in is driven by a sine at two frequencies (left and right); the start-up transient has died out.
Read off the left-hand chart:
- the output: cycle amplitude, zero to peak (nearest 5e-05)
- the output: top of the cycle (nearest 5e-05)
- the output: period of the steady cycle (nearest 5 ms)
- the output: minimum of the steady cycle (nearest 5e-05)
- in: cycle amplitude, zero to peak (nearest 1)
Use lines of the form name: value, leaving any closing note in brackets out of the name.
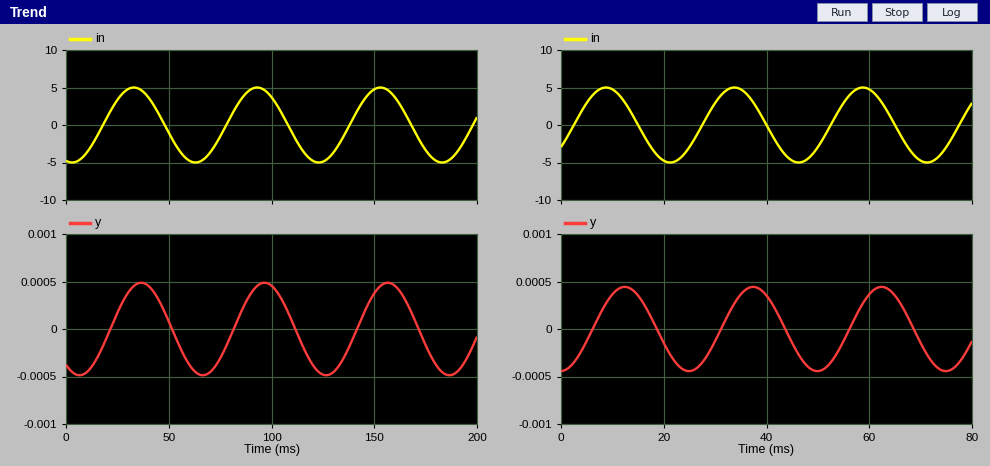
the output: cycle amplitude, zero to peak: 0.00050
the output: top of the cycle: 0.00050
the output: period of the steady cycle: 60 ms
the output: minimum of the steady cycle: -0.00050
in: cycle amplitude, zero to peak: 5
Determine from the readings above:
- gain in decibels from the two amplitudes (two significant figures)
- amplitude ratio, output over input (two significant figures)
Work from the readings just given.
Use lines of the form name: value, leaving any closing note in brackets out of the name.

gain in decibels from the two amplitudes: -80 dB
amplitude ratio, output over input: 0.00010
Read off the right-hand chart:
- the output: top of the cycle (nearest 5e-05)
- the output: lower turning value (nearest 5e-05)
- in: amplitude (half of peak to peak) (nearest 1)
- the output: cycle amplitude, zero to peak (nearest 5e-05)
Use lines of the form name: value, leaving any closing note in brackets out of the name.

the output: top of the cycle: 0.00045
the output: lower turning value: -0.00045
in: amplitude (half of peak to peak): 5
the output: cycle amplitude, zero to peak: 0.00045
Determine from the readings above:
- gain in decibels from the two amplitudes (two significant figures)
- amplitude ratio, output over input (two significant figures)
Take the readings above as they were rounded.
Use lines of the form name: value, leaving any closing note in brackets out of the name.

gain in decibels from the two amplitudes: -81 dB
amplitude ratio, output over input: 0.000090
